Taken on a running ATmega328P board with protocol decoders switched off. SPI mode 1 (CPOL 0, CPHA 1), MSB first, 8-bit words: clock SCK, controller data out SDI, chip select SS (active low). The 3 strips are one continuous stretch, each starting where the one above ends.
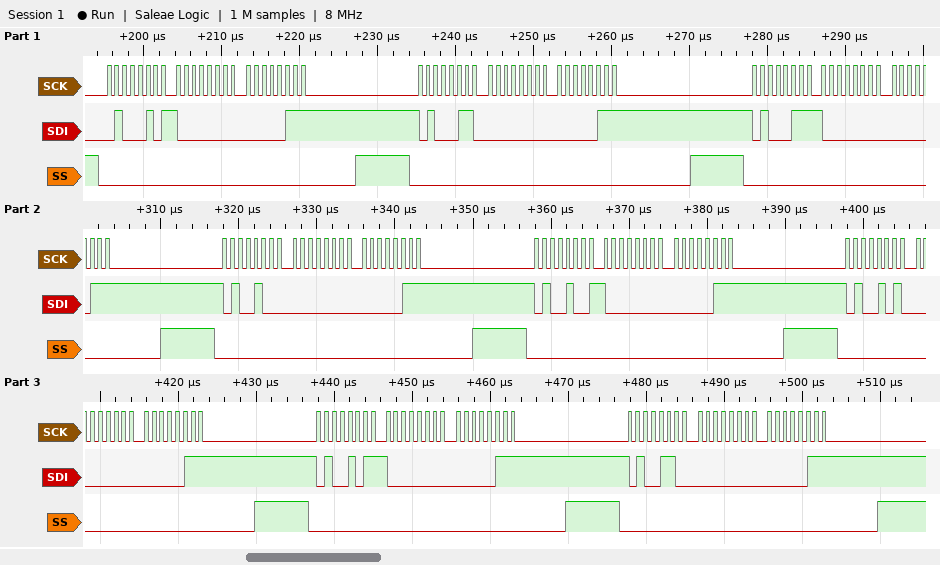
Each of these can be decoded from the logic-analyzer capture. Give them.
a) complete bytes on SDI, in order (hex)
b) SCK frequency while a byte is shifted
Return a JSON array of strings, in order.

["45 00 07 46 00 07 47 00 07 48 00 07 49 00 07 4A 00 07 4B 00 07 4C 00 07", "1 MHz"]
